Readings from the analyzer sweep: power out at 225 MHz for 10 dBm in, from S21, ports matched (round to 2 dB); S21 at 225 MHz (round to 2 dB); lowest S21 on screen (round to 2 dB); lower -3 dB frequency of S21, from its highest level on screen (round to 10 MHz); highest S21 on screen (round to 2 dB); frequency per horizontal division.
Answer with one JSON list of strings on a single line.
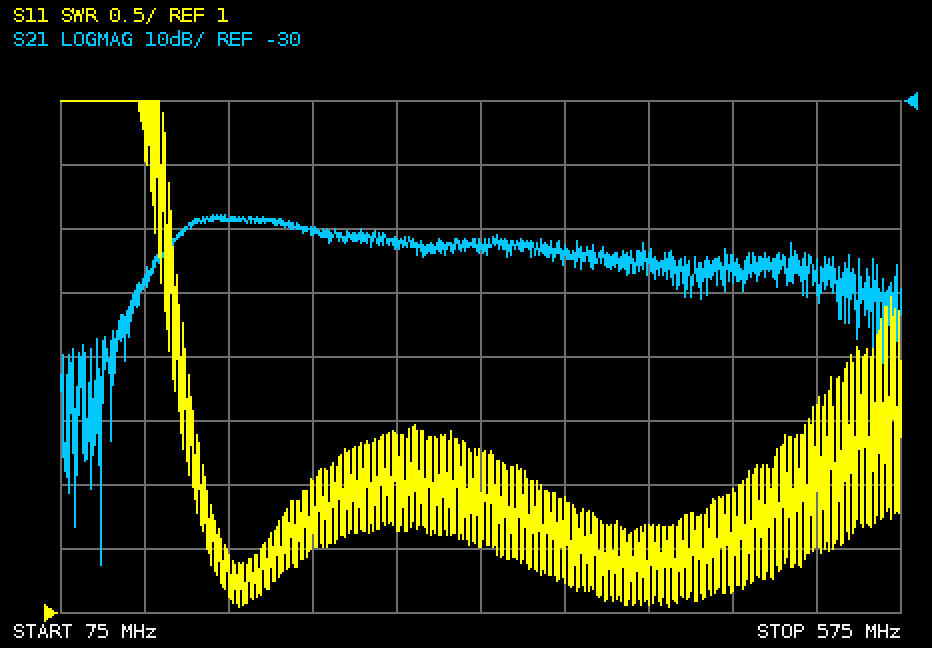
["-40 dBm", "-50 dB", "-102 dB", "150 MHz", "-48 dB", "50 MHz"]
